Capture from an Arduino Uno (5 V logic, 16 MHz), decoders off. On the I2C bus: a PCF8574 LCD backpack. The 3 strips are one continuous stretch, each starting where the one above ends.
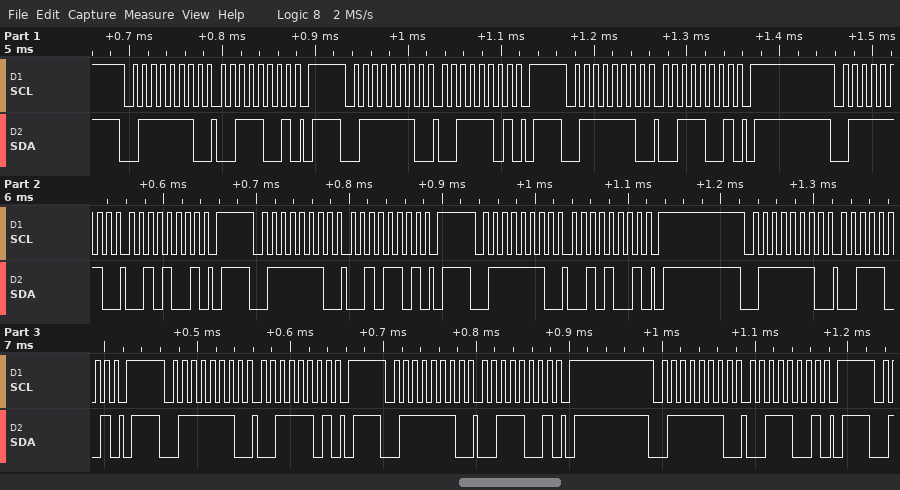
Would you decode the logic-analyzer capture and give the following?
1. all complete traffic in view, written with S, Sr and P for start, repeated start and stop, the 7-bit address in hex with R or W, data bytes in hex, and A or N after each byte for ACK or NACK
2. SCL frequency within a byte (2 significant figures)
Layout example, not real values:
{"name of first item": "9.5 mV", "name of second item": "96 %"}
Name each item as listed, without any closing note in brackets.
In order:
{"all complete traffic in view, written with S, Sr and P for start, repeated start and stop, the 7-bit address in hex with R or W, data bytes in hex, and A or N after each byte for ACK or NACK": "S 3FW A 39 A P S 3FW A 3D A P S 3FW A 39 A P S 3FW A 29 A P S 3FW A 2D A P S 3FW A 29 A P S 3FW A 39 A P S 3FW A 3D A P S 3FW A 39 A P S 3FW A 39 A P", "SCL frequency within a byte": "100 kHz"}
